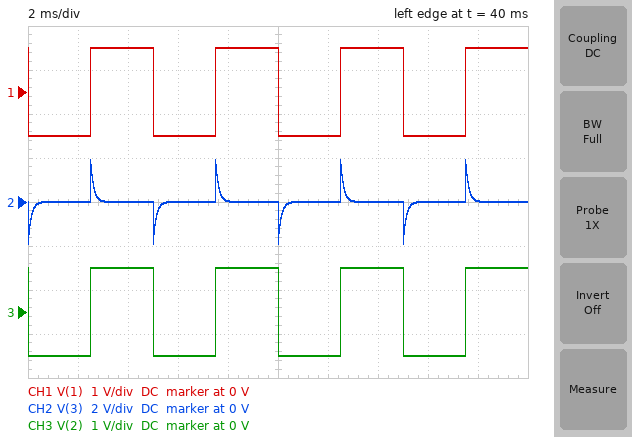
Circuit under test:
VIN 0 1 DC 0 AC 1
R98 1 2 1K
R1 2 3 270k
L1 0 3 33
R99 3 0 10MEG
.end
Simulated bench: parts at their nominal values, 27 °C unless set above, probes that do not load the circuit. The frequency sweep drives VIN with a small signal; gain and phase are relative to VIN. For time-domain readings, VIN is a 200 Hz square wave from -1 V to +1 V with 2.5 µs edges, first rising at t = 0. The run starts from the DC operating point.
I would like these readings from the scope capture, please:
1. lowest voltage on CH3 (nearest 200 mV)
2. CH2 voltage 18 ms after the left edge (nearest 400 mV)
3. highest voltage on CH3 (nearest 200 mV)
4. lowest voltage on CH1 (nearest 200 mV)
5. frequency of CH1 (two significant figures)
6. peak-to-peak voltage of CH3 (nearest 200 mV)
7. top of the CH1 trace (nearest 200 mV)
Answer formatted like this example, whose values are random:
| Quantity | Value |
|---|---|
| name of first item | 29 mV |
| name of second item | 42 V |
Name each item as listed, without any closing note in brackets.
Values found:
| Quantity | Value |
|---|---|
| lowest voltage on CH3 | -1.0 V |
| CH2 voltage 18 ms after the left edge | 0 V |
| highest voltage on CH3 | 1.0 V |
| lowest voltage on CH1 | -1.0 V |
| frequency of CH1 | 200 Hz |
| peak-to-peak voltage of CH3 | 2.0 V |
| top of the CH1 trace | 1.0 V |
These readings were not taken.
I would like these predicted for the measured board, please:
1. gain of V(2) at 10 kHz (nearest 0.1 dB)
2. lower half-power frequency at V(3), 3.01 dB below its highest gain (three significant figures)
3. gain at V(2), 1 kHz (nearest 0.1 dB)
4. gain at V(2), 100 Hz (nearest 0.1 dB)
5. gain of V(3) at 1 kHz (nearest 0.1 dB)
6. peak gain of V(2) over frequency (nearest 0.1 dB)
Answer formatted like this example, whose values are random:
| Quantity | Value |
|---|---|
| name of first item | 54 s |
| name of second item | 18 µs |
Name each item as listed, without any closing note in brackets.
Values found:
| Quantity | Value |
|---|---|
| gain of V(2) at 10 kHz | 0 dB |
| lower half-power frequency at V(3), 3.01 dB below its highest gain | 1.27 kHz |
| gain at V(2), 1 kHz | 0 dB |
| gain at V(2), 100 Hz | 0 dB |
| gain of V(3) at 1 kHz | -4.4 dB |
| peak gain of V(2) over frequency | 0 dB |
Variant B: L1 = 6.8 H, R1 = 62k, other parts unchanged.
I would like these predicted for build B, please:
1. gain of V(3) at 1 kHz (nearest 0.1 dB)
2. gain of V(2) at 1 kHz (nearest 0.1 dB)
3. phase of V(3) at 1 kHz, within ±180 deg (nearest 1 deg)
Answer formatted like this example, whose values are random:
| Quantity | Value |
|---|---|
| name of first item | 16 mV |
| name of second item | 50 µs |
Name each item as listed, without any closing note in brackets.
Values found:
| Quantity | Value |
|---|---|
| gain of V(3) at 1 kHz | -5.0 dB |
| gain of V(2) at 1 kHz | -0.1 dB |
| phase of V(3) at 1 kHz, within ±180 deg | -124 deg |
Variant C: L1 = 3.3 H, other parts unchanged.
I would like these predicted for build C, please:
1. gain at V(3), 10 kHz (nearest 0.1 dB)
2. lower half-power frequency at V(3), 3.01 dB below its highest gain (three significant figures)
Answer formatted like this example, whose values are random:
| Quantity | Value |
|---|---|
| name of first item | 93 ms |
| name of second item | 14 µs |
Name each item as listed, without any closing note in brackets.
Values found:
| Quantity | Value |
|---|---|
| gain at V(3), 10 kHz | -4.4 dB |
| lower half-power frequency at V(3), 3.01 dB below its highest gain | 12.7 kHz |
